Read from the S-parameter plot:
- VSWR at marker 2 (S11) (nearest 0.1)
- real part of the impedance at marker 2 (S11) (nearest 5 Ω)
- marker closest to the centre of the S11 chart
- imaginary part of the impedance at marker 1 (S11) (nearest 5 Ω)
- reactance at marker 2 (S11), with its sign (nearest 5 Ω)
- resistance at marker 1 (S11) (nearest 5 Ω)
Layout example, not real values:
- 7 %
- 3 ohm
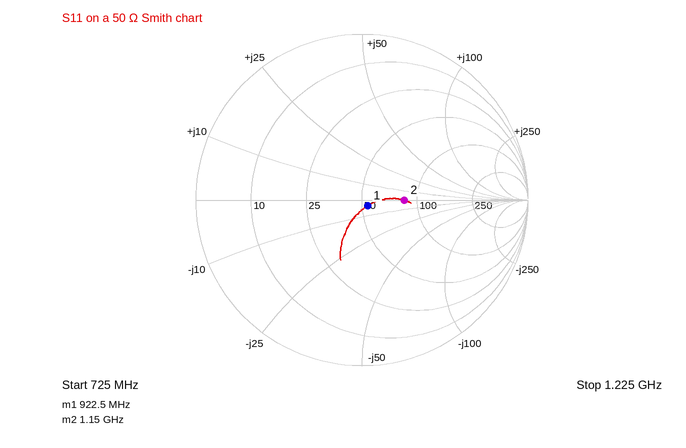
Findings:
- 1.7
- 85 Ω
- marker 1
- -5 Ω
- 0 Ω
- 55 Ω
